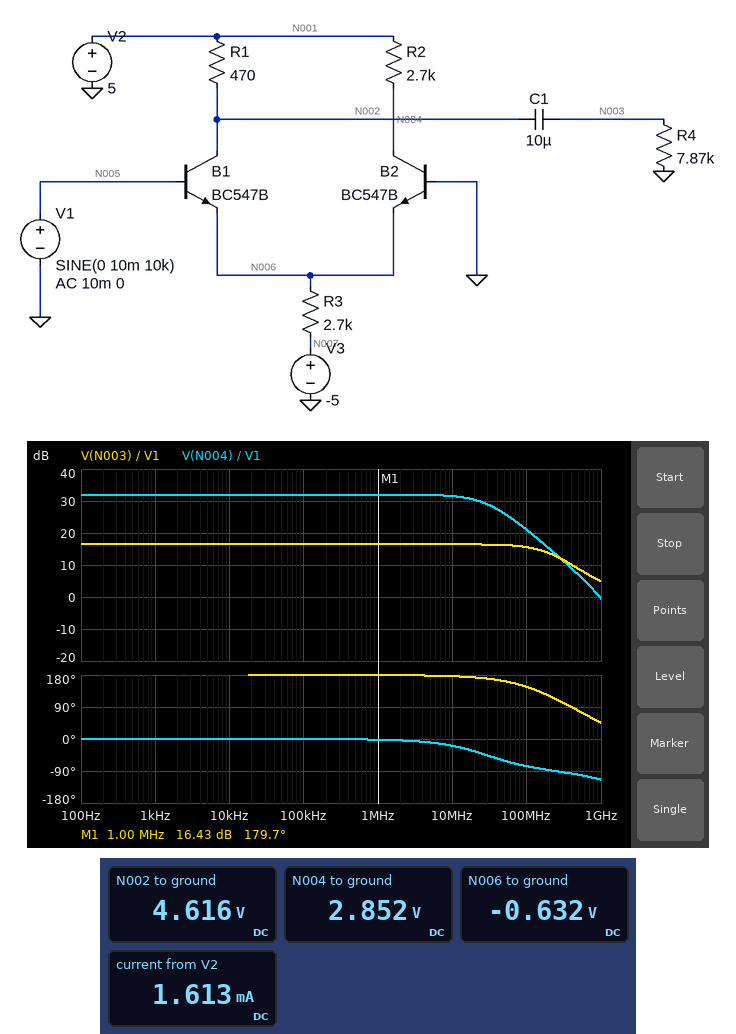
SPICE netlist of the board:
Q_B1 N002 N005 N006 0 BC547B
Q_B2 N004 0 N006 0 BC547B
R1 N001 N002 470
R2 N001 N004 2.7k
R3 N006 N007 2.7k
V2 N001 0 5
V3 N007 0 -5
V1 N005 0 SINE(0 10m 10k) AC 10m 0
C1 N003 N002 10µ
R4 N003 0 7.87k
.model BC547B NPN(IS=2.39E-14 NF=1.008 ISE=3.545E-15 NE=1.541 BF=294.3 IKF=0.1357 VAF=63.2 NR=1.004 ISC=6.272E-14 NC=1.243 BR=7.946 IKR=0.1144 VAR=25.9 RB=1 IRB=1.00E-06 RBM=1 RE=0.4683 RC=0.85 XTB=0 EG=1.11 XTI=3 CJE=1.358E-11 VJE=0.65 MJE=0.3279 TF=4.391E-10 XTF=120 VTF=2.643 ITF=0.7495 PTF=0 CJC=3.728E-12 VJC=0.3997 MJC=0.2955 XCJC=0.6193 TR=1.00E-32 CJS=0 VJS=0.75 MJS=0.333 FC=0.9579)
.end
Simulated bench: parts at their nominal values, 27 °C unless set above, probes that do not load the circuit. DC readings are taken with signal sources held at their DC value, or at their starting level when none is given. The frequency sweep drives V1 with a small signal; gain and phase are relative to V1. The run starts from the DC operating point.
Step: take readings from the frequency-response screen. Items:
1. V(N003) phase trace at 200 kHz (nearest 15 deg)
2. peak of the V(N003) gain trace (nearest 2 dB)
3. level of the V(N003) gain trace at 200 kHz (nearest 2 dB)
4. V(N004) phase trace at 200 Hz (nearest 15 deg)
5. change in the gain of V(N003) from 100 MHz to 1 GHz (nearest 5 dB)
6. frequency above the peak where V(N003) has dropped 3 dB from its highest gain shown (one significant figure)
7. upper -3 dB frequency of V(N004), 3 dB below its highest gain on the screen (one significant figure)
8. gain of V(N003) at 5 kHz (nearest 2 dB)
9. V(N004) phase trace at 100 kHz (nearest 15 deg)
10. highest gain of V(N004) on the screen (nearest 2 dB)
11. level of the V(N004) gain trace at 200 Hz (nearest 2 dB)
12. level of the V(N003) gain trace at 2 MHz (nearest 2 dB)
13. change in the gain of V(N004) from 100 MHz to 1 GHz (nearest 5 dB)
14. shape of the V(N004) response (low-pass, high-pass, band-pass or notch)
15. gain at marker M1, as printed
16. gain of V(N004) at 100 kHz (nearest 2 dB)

180 deg
16 dB
16 dB
0 deg
-10 dB
200 MHz
30 MHz
16 dB
0 deg
32 dB
32 dB
16 dB
-20 dB
low-pass
16.43 dB
32 dB
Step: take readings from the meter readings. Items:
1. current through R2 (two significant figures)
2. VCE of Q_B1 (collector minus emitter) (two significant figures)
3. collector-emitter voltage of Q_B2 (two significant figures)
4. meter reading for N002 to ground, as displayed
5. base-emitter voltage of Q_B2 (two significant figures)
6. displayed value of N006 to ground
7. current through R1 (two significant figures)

800 µA
5.2 V
3.5 V
4.616 V
630 mV
-0.632 V
820 µA
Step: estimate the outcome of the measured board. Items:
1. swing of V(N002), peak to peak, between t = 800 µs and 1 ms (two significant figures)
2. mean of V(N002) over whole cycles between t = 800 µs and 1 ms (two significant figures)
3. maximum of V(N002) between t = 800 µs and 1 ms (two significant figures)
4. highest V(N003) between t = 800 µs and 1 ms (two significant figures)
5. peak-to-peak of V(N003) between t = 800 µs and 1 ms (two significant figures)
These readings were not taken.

130 mV
4.6 V
4.7 V
66 mV
130 mV
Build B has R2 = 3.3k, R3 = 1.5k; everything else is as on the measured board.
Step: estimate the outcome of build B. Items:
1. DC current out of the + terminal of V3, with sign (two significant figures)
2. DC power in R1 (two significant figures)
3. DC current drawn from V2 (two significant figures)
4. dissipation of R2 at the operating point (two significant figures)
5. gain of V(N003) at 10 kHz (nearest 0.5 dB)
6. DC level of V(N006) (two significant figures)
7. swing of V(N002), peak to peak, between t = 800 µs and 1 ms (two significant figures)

-2.9 mA
1.0 mW
2.9 mA
6.5 mW
21.0 dB
-650 mV
230 mV
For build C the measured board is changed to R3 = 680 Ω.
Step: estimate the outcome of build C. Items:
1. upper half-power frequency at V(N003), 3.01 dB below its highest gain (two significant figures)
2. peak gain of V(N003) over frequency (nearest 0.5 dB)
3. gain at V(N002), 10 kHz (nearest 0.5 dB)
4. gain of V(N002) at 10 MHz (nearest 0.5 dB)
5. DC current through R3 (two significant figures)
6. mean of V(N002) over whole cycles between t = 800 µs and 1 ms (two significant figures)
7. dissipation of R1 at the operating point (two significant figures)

250 MHz
28.0 dB
18.0 dB
19.5 dB
6.4 mA
3.1 V
7.5 mW
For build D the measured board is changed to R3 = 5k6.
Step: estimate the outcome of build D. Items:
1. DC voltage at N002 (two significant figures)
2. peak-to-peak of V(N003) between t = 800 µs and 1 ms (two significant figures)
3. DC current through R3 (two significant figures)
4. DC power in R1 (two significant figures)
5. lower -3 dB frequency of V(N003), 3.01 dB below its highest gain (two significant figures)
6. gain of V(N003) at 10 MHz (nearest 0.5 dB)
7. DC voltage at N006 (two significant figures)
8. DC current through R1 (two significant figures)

4.8 V
65 mV
780 µA
73 µW
1.9 Hz
10.5 dB
-610 mV
390 µA
